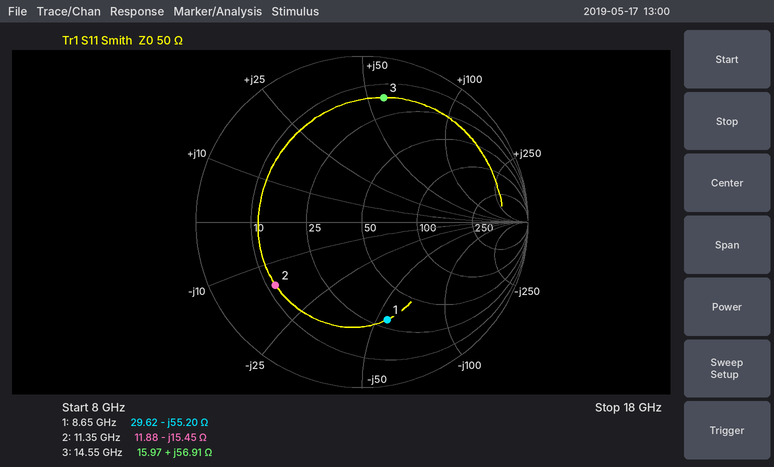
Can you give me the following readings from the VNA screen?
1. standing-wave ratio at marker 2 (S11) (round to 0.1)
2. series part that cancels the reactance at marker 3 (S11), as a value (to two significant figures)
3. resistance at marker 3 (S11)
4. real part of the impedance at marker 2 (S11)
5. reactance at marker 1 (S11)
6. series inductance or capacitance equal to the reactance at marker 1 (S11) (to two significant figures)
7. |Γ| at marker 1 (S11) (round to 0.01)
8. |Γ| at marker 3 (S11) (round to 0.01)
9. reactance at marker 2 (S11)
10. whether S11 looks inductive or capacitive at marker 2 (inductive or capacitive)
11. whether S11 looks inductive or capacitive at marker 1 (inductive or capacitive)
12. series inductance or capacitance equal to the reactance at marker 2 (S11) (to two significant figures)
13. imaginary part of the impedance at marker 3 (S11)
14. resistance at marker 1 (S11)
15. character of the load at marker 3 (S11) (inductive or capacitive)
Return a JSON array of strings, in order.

["4.6", "190 fF", "15.97 Ω", "11.88 Ω", "-55.20 Ω", "330 fF", "0.61", "0.76", "-15.45 Ω", "capacitive", "capacitive", "910 fF", "+56.91 Ω", "29.62 Ω", "inductive"]
